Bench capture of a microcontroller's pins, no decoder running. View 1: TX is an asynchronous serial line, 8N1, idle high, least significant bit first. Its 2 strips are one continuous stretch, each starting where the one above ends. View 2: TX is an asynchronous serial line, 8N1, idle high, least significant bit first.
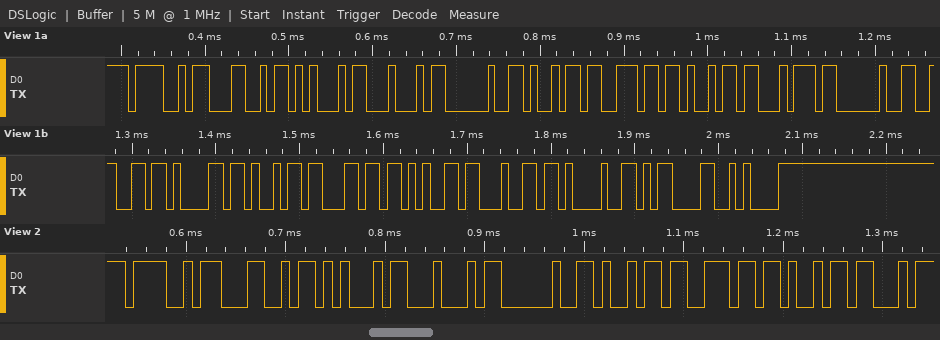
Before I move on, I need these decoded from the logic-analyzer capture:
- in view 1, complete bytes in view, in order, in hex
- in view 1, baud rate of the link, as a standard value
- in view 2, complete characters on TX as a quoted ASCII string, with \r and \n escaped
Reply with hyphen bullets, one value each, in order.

- 0x4F 0x4C 0x45 0x44 0x20 0x69 0x6E 0x69 0x74 0x20 0x66 0x61 0x69 0x6C 0x65 0x64 0x21 0x0D 0x0A
- 115200 baud
- "OLED ini"
